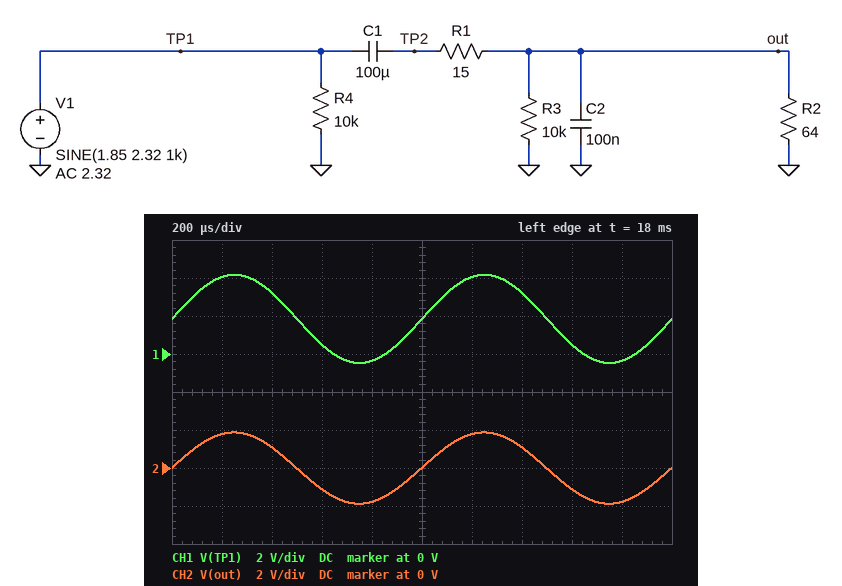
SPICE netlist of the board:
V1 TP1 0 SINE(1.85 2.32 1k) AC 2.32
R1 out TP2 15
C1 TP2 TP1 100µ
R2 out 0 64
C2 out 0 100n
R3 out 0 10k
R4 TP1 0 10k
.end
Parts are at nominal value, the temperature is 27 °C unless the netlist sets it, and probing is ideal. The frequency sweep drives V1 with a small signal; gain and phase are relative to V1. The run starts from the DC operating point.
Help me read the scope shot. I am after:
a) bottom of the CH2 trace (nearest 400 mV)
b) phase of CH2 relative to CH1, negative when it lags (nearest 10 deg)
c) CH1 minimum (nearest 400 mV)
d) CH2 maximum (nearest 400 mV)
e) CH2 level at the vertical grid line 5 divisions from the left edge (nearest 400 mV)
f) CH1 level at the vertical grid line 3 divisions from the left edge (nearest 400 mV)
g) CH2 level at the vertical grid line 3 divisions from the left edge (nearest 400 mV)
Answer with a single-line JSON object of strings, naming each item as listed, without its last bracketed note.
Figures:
{"bottom of the CH2 trace": "-2.0 V", "phase of CH2 relative to CH1, negative when it lags": "0 deg", "CH1 minimum": "-400 mV", "CH2 maximum": "2.0 V", "CH2 level at the vertical grid line 5 divisions from the left edge": "0 V", "CH1 level at the vertical grid line 3 divisions from the left edge": "400 mV", "CH2 level at the vertical grid line 3 divisions from the left edge": "-1.2 V"}
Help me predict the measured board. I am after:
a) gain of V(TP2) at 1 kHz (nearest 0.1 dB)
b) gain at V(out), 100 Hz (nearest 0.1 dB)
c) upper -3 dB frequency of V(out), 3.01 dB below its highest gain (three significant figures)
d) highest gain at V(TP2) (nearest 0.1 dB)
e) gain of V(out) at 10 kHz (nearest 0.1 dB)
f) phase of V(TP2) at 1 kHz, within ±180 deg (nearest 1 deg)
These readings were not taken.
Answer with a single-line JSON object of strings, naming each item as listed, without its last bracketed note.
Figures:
{"gain of V(TP2) at 1 kHz": "0 dB", "gain at V(out), 100 Hz": "-2.0 dB", "upper -3 dB frequency of V(out), 3.01 dB below its highest gain": "131 kHz", "highest gain at V(TP2)": "0 dB", "gain of V(out) at 10 kHz": "-1.9 dB", "phase of V(TP2) at 1 kHz, within ±180 deg": "1 deg"}
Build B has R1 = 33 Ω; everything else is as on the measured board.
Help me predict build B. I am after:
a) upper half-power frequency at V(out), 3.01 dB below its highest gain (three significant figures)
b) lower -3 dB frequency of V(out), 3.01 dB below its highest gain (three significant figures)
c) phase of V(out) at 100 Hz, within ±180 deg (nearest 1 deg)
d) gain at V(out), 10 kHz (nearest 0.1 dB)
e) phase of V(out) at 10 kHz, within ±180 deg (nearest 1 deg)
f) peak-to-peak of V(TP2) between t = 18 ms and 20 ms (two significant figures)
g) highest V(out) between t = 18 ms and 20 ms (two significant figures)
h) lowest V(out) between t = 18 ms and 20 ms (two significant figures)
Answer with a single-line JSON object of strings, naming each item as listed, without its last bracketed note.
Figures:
{"upper half-power frequency at V(out), 3.01 dB below its highest gain": "73.3 kHz", "lower -3 dB frequency of V(out), 3.01 dB below its highest gain": "16.5 Hz", "phase of V(out) at 100 Hz, within ±180 deg": "9 deg", "gain at V(out), 10 kHz": "-3.7 dB", "phase of V(out) at 10 kHz, within ±180 deg": "-8 deg", "peak-to-peak of V(TP2) between t = 18 ms and 20 ms": "4.6 V", "highest V(out) between t = 18 ms and 20 ms": "1.5 V", "lowest V(out) between t = 18 ms and 20 ms": "-1.5 V"}
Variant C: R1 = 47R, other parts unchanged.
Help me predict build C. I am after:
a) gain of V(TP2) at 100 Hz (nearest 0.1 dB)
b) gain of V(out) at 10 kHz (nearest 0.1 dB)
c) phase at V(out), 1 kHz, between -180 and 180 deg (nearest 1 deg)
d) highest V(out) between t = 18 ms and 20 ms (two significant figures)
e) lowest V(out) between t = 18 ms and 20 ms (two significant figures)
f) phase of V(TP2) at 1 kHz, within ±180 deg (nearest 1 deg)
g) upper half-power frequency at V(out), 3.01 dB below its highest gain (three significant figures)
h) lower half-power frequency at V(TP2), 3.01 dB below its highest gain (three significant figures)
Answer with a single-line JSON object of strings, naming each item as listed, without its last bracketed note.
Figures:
{"gain of V(TP2) at 100 Hz": "-0.1 dB", "gain of V(out) at 10 kHz": "-4.9 dB", "phase at V(out), 1 kHz, between -180 and 180 deg": "0 deg", "highest V(out) between t = 18 ms and 20 ms": "1.3 V", "lowest V(out) between t = 18 ms and 20 ms": "-1.3 V", "phase of V(TP2) at 1 kHz, within ±180 deg": "1 deg", "upper half-power frequency at V(out), 3.01 dB below its highest gain": "58.9 kHz", "lower half-power frequency at V(TP2), 3.01 dB below its highest gain": "14.4 Hz"}
